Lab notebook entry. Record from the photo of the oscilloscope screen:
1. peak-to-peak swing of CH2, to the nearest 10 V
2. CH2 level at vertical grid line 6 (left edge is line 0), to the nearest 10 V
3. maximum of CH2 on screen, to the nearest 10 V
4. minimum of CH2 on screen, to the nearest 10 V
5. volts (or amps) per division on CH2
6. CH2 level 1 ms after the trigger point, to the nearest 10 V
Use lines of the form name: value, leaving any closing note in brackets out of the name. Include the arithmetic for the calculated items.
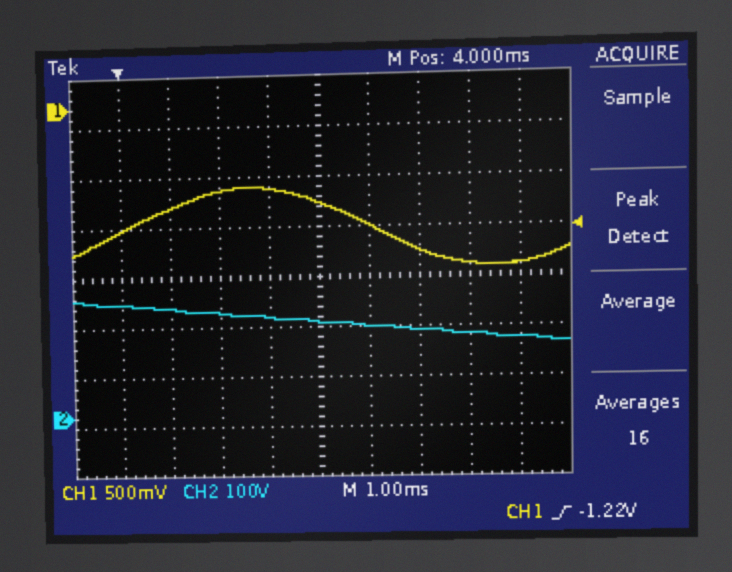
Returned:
peak-to-peak swing of CH2, to the nearest 10 V: 240 V − (150 V) = 90 V
CH2 level at vertical grid line 6 (left edge is line 0), to the nearest 10 V: 180 V
maximum of CH2 on screen, to the nearest 10 V: 240 V
minimum of CH2 on screen, to the nearest 10 V: 150 V
volts (or amps) per division on CH2: 100 V
CH2 level 1 ms after the trigger point, to the nearest 10 V: 220 V
